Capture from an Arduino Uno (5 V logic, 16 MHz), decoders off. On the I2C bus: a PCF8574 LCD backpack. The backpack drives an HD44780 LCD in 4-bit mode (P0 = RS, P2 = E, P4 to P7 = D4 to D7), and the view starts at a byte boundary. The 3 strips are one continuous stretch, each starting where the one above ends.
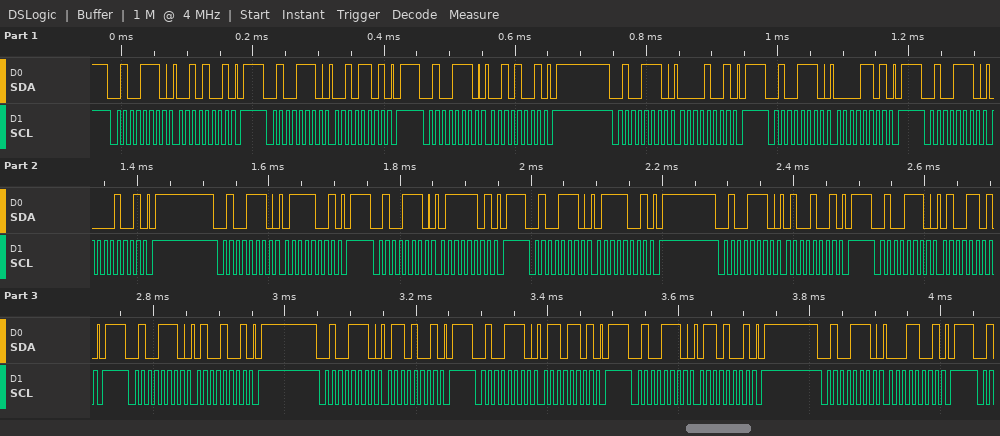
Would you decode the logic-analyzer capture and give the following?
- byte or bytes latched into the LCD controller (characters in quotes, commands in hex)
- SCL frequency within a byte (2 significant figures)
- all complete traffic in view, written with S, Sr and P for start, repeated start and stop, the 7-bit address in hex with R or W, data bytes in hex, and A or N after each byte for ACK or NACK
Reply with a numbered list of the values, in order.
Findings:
1. ' ' 't'
2. 100 kHz
3. S 27W A 29 A P S 27W A 2D A P S 27W A 29 A P S 27W A 09 A P S 27W A 0D A P S 27W A 09 A P S 27W A 79 A P S 27W A 7D A P S 27W A 79 A P S 27W A 49 A P S 27W A 4D A P S 27W A 49 A P S 27W A 69 A P S 27W A 6D A P S 27W A 69 A P S 27W A 19 A P
